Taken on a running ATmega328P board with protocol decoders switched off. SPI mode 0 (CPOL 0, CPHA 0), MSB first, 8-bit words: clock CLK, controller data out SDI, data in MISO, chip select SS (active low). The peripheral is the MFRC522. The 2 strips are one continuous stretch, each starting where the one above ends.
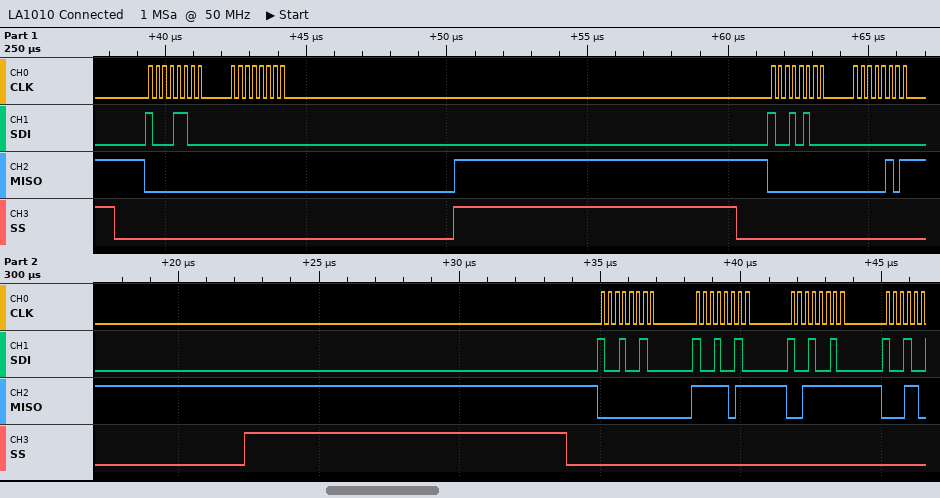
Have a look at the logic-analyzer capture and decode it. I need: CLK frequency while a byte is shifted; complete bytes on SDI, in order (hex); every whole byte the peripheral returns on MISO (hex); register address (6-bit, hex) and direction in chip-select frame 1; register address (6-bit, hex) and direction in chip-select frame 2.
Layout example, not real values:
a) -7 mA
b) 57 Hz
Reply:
a) 4 MHz
b) 8C 00 94 00 92 92 92
c) 00 00 00 05 00 FB 3F
d) 0x06 read
e) 0x0A read
